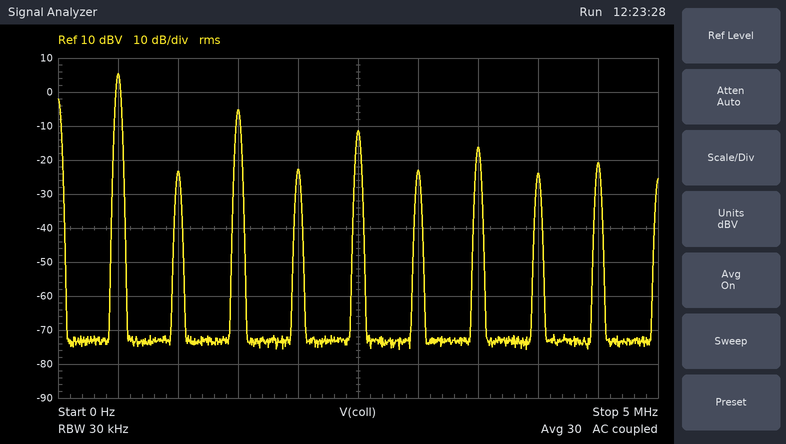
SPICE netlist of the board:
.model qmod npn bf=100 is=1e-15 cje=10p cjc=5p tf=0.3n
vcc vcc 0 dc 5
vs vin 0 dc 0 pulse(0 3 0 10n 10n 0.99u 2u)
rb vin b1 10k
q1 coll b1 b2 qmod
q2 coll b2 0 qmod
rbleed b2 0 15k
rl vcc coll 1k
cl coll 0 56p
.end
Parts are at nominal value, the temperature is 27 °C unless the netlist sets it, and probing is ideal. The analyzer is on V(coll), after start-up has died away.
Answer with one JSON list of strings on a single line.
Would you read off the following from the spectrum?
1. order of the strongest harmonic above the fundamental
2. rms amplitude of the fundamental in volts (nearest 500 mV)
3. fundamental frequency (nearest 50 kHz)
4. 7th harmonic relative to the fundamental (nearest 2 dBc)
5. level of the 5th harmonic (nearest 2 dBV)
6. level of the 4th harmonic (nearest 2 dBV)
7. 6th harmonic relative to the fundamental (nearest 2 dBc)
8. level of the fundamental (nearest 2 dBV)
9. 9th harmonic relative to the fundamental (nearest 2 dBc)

["3", "2.0 V", "500 kHz", "-22 dBc", "-12 dBV", "-22 dBV", "-28 dBc", "6 dBV", "-26 dBc"]
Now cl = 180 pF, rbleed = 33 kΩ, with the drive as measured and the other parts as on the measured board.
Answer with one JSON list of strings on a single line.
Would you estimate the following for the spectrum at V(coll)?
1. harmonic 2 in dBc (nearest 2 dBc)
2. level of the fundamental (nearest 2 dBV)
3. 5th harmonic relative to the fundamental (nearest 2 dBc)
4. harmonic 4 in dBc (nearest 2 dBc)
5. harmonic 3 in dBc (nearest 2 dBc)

["-18 dBc", "4 dBV", "-18 dBc", "-22 dBc", "-12 dBc"]
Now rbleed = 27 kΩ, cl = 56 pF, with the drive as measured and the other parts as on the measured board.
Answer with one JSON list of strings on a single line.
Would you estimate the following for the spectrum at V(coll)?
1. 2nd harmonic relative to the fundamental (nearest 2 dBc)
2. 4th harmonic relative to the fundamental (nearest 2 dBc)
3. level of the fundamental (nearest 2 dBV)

["-26 dBc", "-26 dBc", "6 dBV"]
